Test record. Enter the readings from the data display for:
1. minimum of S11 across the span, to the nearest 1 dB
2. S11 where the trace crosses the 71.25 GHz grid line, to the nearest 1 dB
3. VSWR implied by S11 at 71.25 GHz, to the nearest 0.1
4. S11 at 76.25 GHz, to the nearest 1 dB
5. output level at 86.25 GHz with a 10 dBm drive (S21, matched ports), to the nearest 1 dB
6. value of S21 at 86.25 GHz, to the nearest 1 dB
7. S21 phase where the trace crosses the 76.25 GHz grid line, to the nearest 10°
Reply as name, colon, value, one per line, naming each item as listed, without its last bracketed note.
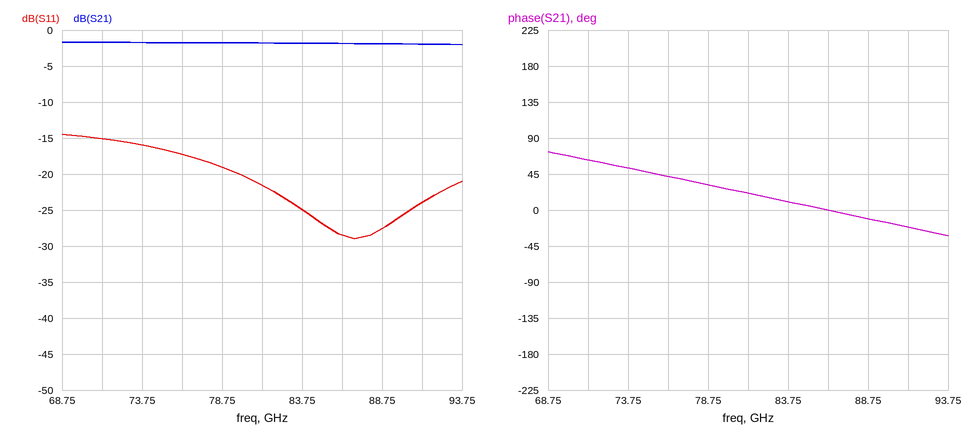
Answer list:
minimum of S11 across the span, to the nearest 1 dB: -29 dB
S11 where the trace crosses the 71.25 GHz grid line, to the nearest 1 dB: -15 dB
VSWR implied by S11 at 71.25 GHz, to the nearest 0.1: 1.4
S11 at 76.25 GHz, to the nearest 1 dB: -17 dB
output level at 86.25 GHz with a 10 dBm drive (S21, matched ports), to the nearest 1 dB: 8 dBm
value of S21 at 86.25 GHz, to the nearest 1 dB: -2 dB
S21 phase where the trace crosses the 76.25 GHz grid line, to the nearest 10°: 40°
